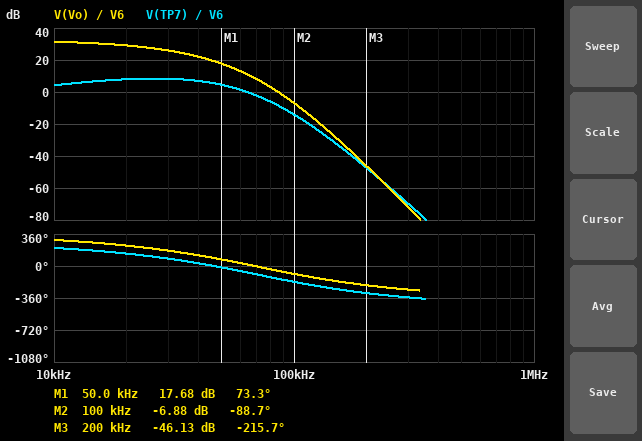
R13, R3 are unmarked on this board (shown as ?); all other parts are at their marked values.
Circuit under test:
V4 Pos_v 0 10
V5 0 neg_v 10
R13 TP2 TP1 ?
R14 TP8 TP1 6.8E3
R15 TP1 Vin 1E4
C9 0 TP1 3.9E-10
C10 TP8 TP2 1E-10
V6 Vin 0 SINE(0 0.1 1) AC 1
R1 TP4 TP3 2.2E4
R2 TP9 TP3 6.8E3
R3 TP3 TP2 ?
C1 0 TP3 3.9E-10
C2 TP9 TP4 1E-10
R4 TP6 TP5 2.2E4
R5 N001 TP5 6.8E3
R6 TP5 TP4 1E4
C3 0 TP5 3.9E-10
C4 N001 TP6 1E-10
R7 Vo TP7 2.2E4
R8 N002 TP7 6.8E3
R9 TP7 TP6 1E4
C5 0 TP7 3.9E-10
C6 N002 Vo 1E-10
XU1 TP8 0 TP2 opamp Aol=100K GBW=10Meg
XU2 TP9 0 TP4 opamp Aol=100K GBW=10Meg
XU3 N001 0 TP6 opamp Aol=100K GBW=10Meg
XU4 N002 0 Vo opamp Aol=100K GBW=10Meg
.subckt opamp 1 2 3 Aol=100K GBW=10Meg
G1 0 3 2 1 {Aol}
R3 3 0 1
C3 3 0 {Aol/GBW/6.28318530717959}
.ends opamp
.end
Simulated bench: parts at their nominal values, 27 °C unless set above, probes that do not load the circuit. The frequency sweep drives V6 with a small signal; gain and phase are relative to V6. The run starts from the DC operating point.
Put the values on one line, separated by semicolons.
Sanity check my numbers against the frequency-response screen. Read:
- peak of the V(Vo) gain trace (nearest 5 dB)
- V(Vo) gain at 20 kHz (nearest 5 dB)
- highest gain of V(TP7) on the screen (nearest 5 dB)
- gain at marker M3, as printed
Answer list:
30 dB; 30 dB; 10 dB; -46.13 dB
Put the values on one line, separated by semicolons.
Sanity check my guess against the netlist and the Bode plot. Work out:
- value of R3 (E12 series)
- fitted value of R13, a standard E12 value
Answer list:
3.9 kΩ; 15 kΩ
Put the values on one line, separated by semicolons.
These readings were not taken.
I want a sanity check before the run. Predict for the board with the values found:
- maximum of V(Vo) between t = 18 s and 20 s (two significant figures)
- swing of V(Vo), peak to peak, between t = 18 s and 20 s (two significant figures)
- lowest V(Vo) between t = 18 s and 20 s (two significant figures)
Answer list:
4.1 V; 8.2 V; -4.1 V
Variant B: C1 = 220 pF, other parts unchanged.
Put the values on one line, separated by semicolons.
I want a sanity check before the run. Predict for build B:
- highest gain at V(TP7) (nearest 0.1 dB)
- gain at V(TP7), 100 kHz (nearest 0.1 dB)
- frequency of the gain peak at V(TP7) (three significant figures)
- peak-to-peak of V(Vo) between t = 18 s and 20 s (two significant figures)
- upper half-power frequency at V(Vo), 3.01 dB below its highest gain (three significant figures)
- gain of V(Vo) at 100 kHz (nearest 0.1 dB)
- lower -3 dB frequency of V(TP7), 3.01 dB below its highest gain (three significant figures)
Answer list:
8.1 dB; -13.7 dB; 25.9 kHz; 8.2 V; 18.9 kHz; -6.5 dB; 11.6 kHz
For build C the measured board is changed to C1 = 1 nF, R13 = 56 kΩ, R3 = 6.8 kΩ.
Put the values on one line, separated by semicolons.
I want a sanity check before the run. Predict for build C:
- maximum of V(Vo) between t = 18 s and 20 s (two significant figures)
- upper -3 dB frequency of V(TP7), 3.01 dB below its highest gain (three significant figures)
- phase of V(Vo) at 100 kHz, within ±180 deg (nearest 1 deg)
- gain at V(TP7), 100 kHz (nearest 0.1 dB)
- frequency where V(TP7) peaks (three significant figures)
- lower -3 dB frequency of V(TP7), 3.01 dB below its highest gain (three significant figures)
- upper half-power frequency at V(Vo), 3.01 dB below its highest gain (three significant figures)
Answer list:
8.8 V; 37.1 kHz; -150 deg; -21.6 dB; 21.8 kHz; 9.88 kHz; 15.9 kHz
